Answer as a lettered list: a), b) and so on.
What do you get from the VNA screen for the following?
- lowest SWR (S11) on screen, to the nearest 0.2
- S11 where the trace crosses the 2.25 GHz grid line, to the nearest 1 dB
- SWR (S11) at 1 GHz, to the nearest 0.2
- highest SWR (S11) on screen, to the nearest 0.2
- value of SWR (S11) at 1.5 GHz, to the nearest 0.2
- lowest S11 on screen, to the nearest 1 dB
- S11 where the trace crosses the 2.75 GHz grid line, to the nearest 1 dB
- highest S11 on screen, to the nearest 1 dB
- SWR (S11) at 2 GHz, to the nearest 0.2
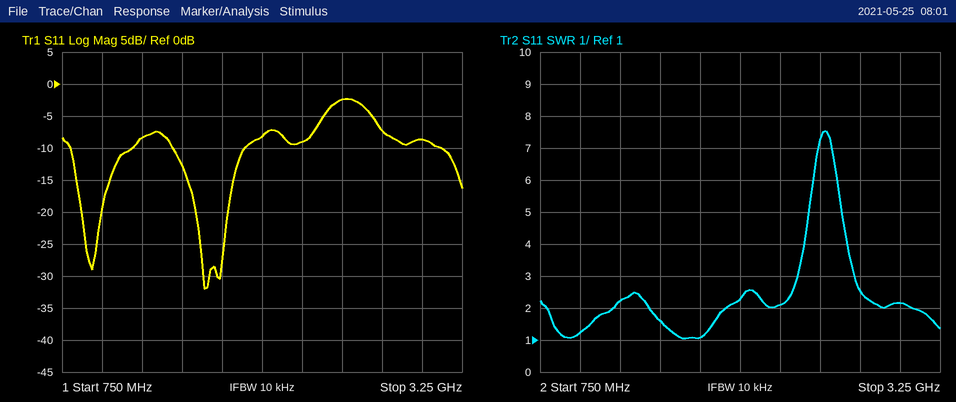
a) 1.0
b) -9 dB
c) 1.2
d) 7.6
e) 1.6
f) -32 dB
g) -7 dB
h) -2 dB
i) 2.2
